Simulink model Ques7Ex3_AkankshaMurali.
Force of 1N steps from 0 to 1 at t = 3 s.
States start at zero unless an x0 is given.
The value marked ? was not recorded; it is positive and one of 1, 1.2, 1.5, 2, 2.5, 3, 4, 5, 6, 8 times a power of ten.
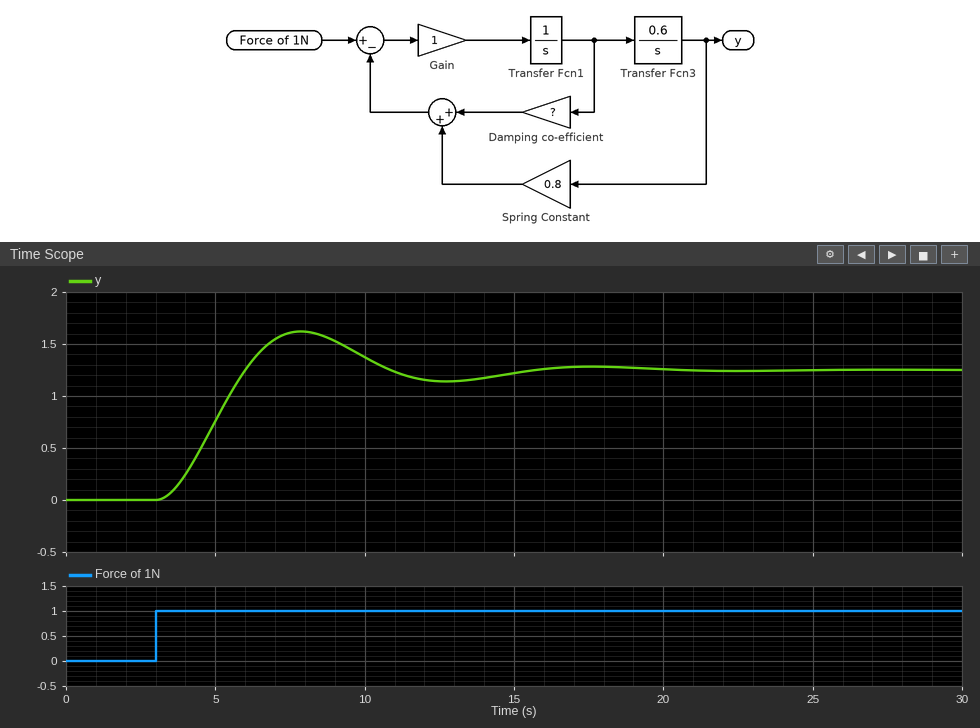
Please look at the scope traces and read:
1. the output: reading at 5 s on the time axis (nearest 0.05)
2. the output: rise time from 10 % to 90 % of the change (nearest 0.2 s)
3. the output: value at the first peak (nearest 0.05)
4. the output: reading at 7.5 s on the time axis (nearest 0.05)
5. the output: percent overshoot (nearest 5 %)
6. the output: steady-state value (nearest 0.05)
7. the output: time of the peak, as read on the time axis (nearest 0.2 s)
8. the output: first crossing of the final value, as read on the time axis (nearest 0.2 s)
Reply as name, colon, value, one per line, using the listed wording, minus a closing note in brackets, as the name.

the output: reading at 5 s on the time axis: 0.75
the output: rise time from 10 % to 90 % of the change: 2.0 s
the output: value at the first peak: 1.60
the output: reading at 7.5 s on the time axis: 1.60
the output: percent overshoot: 30 %
the output: steady-state value: 1.25
the output: time of the peak, as read on the time axis: 7.8 s
the output: first crossing of the final value, as read on the time axis: 6.0 s
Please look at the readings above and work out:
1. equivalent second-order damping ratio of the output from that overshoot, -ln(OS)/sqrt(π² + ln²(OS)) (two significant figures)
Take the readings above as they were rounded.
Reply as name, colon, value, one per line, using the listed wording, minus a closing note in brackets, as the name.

equivalent second-order damping ratio of the output from that overshoot, -ln(OS)/sqrt(π² + ln²(OS)): 0.36
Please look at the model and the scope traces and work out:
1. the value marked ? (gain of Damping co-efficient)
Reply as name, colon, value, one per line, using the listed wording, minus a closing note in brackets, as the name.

the value marked ?: 0.5
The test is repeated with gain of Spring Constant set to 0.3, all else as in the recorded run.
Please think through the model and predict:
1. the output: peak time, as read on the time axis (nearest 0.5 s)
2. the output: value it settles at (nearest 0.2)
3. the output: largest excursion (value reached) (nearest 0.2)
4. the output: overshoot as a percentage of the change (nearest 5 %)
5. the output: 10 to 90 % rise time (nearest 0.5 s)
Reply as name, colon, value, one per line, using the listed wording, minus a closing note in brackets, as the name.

the output: peak time, as read on the time axis: 12.0 s
the output: value it settles at: 3.4
the output: largest excursion (value reached): 3.6
the output: overshoot as a percentage of the change: 10 %
the output: 10 to 90 % rise time: 4.5 s
